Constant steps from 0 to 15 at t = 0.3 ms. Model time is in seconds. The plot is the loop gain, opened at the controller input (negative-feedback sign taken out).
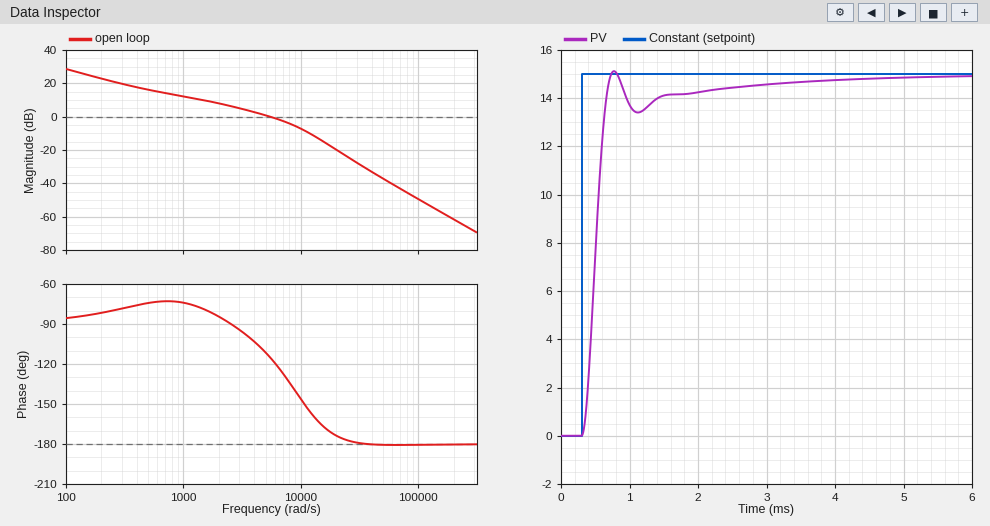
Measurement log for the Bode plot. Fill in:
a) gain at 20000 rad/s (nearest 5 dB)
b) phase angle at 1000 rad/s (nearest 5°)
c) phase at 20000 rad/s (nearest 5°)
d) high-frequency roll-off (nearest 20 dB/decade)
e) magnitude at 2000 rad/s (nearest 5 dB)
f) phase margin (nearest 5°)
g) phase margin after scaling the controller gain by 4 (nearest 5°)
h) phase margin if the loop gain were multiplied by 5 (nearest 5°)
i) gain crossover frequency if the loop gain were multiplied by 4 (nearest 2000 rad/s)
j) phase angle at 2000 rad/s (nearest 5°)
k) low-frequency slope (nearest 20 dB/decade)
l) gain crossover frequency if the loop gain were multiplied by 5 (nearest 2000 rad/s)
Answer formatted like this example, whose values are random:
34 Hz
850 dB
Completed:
-20 dB
-75°
-175°
-40 dB/decade
10 dB
65°
20°
15°
14000 rad/s
-85°
-20 dB/decade
14000 rad/s
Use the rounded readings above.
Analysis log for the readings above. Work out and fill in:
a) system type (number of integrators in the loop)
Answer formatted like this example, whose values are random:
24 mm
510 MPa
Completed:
1
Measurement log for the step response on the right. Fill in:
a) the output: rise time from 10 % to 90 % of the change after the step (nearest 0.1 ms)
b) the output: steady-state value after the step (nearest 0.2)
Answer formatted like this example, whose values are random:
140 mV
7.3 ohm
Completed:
0.3 ms
15.0
